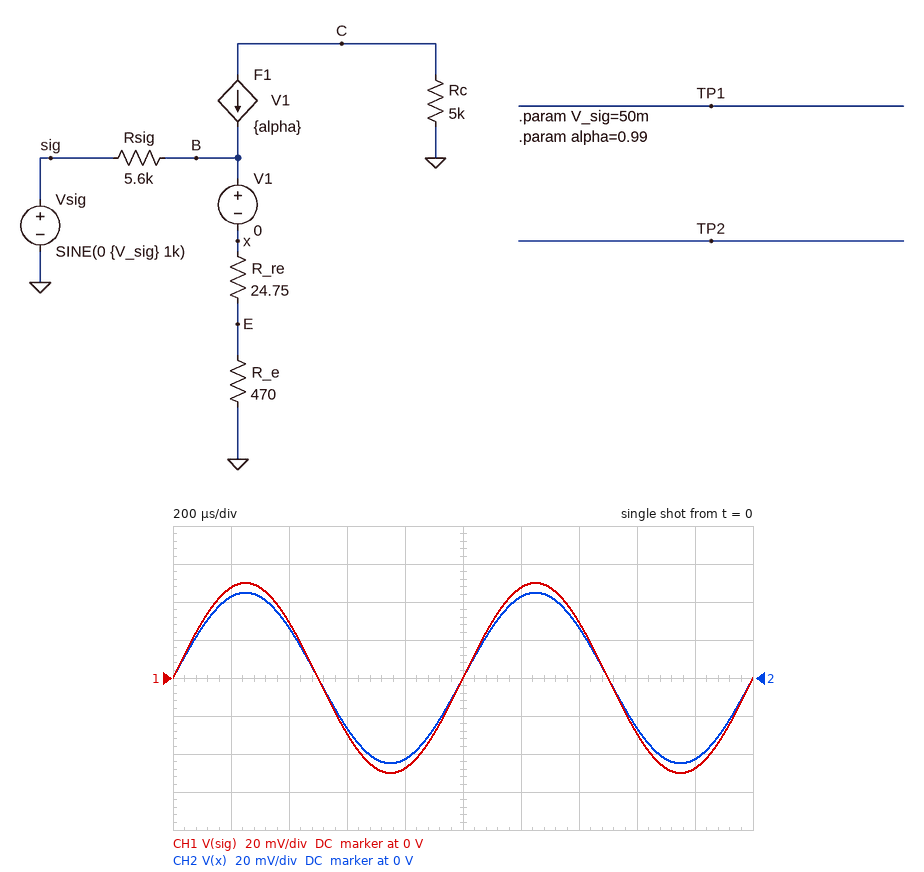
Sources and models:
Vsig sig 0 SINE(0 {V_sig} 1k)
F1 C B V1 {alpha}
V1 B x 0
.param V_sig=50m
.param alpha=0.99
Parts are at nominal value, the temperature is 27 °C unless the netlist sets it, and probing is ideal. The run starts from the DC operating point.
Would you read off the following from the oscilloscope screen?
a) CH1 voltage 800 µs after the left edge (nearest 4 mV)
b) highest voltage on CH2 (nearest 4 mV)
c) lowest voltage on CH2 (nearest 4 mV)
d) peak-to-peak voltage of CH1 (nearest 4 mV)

-48 mV
44 mV
-44 mV
100 mV
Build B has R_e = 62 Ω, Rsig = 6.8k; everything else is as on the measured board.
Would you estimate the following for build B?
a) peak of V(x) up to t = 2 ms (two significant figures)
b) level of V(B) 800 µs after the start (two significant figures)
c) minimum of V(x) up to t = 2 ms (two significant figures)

28 mV
-27 mV
-28 mV
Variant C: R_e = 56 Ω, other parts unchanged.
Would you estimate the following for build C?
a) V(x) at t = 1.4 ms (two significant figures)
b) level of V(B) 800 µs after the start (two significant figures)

17 mV
-28 mV
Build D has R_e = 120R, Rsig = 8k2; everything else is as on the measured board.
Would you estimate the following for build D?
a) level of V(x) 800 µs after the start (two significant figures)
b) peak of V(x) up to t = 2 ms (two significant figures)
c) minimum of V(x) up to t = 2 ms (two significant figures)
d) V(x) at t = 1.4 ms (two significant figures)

-30 mV
32 mV
-32 mV
19 mV
